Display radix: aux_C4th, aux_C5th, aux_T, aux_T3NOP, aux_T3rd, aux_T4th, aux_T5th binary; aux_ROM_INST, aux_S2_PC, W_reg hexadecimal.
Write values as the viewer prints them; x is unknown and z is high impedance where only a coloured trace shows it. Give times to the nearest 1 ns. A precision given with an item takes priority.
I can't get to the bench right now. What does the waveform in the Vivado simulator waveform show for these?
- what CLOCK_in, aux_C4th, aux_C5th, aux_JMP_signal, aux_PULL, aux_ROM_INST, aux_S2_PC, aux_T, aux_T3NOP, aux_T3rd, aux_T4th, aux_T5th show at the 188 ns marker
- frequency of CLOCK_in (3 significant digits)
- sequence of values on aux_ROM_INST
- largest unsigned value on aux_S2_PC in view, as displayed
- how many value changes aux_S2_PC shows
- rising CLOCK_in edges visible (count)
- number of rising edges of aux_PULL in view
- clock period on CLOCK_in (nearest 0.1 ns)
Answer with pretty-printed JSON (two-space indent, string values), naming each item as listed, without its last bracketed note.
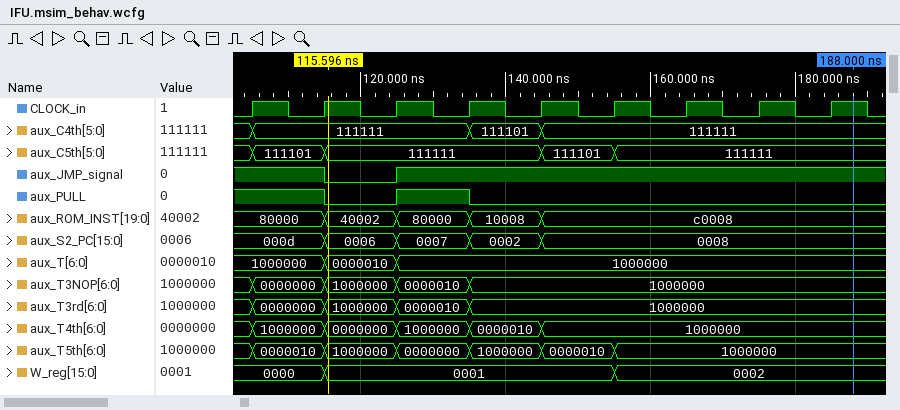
{
  "what CLOCK_in, aux_C4th, aux_C5th, aux_JMP_signal, aux_PULL, aux_ROM_INST, aux_S2_PC, aux_T, aux_T3NOP, aux_T3rd, aux_T4th, aux_T5th show at the 188 ns marker": "CLOCK_in=1, aux_C4th=111111, aux_C5th=111111, aux_JMP_signal=1, aux_PULL=0, aux_ROM_INST=c0008, aux_S2_PC=0008, aux_T=1000000, aux_T3NOP=1000000, aux_T3rd=1000000, aux_T4th=1000000, aux_T5th=1000000",
  "frequency of CLOCK_in": "100 MHz",
  "sequence of values on aux_ROM_INST": "80000, 40002, 80000, 10008, c0008",
  "largest unsigned value on aux_S2_PC in view, as displayed": "000d",
  "how many value changes aux_S2_PC shows": "4",
  "rising CLOCK_in edges visible": "9",
  "number of rising edges of aux_PULL in view": "1",
  "clock period on CLOCK_in": "10 ns"
}
